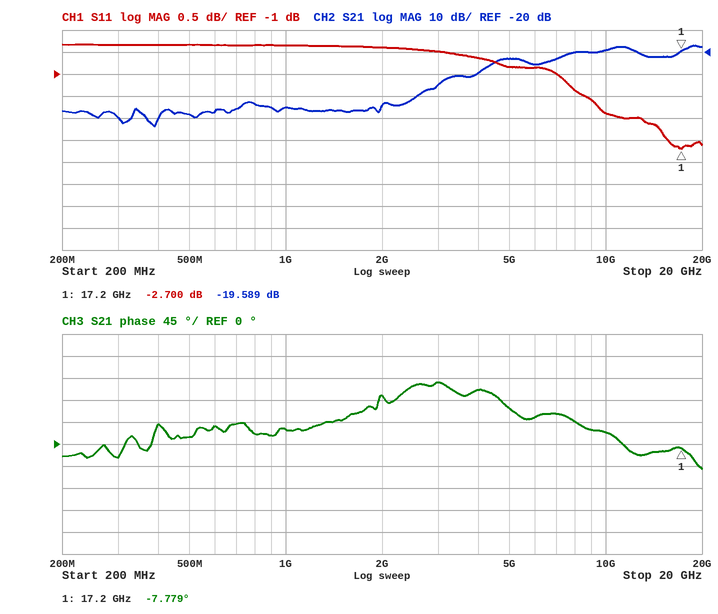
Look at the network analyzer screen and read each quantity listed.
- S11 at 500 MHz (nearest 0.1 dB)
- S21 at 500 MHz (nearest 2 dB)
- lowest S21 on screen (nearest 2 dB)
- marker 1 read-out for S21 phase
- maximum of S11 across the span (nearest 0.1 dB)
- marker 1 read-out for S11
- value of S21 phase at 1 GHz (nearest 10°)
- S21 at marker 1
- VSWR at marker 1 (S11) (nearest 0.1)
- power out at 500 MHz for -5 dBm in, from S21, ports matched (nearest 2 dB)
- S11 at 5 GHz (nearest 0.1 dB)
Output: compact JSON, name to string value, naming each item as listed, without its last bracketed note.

{"S11 at 500 MHz": "-0.3 dB", "S21 at 500 MHz": "-48 dB", "lowest S21 on screen": "-54 dB", "marker 1 read-out for S21 phase": "-7.779°", "maximum of S11 across the span": "-0.3 dB", "marker 1 read-out for S11": "-2.700 dB", "value of S21 phase at 1 GHz": "30°", "S21 at marker 1": "-19.589 dB", "VSWR at marker 1 (S11)": "6.5", "power out at 500 MHz for -5 dBm in, from S21, ports matched": "-54 dBm", "S11 at 5 GHz": "-0.8 dB"}
